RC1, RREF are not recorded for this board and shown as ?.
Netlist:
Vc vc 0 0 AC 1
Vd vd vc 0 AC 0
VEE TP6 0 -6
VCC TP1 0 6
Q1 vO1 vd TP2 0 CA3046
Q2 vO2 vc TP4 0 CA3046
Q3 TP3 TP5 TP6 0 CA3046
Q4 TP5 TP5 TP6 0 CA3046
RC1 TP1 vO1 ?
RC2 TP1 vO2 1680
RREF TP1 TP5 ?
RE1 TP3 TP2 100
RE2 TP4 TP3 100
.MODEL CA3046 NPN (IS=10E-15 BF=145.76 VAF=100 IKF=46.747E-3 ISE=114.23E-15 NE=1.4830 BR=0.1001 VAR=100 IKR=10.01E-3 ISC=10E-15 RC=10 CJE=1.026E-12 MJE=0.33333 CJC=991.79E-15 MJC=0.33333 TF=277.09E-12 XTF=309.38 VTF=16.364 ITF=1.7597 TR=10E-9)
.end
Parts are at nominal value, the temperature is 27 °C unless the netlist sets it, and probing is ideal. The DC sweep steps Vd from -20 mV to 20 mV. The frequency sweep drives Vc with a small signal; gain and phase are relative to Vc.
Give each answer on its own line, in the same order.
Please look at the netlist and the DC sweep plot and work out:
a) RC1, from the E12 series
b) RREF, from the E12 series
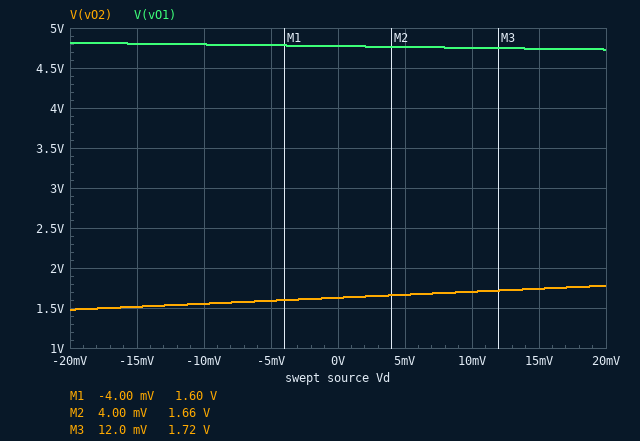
470 Ω
2.2 kΩ
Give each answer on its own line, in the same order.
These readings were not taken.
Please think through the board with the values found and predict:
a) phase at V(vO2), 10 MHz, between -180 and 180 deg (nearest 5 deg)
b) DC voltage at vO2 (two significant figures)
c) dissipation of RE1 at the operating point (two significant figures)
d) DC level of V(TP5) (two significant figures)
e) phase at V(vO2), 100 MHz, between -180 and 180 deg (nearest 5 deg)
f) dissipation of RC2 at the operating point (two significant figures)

155 deg
1.6 V
690 µW
-5.3 V
95 deg
11 mW
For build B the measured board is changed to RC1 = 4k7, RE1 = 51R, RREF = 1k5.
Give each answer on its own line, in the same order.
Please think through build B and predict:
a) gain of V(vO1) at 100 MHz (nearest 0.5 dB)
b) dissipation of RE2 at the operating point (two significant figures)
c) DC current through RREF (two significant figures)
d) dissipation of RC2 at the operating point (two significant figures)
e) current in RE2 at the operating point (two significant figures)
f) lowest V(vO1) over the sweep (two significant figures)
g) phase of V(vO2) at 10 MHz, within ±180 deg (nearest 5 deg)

0 dB
750 µW
7.5 mA
12 mW
2.7 mA
-630 mV
135 deg
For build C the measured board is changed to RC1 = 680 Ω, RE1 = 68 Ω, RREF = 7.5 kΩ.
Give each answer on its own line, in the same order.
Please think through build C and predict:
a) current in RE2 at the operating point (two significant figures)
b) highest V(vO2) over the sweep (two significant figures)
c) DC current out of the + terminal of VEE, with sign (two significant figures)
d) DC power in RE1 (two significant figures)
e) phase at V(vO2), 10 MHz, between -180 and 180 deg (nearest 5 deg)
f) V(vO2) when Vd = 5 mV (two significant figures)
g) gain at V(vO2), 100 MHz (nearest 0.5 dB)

670 µA
5.0 V
-3.1 mA
53 µW
140 deg
4.9 V
-13.5 dB
